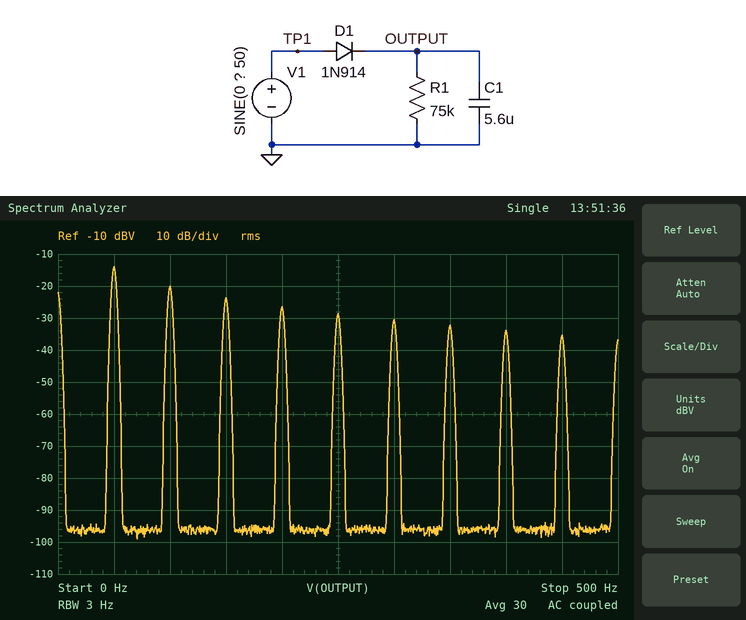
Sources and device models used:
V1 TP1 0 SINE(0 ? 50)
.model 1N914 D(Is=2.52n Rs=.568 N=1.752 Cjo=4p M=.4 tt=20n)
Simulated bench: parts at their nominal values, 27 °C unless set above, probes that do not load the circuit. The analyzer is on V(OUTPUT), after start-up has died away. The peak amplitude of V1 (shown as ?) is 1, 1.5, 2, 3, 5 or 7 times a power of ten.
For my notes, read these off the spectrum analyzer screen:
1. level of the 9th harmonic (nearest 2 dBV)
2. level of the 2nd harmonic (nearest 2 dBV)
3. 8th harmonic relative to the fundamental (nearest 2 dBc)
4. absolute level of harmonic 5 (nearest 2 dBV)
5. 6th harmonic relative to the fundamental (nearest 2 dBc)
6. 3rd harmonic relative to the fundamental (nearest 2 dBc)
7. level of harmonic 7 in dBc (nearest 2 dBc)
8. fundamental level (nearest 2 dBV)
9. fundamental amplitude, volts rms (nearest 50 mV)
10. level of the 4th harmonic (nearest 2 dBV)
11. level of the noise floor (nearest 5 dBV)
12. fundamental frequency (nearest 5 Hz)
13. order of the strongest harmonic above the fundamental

-36 dBV
-20 dBV
-20 dBc
-28 dBV
-16 dBc
-10 dBc
-18 dBc
-14 dBV
200 mV
-26 dBV
-95 dBV
50 Hz
2
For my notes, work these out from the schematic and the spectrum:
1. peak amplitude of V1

20 V
